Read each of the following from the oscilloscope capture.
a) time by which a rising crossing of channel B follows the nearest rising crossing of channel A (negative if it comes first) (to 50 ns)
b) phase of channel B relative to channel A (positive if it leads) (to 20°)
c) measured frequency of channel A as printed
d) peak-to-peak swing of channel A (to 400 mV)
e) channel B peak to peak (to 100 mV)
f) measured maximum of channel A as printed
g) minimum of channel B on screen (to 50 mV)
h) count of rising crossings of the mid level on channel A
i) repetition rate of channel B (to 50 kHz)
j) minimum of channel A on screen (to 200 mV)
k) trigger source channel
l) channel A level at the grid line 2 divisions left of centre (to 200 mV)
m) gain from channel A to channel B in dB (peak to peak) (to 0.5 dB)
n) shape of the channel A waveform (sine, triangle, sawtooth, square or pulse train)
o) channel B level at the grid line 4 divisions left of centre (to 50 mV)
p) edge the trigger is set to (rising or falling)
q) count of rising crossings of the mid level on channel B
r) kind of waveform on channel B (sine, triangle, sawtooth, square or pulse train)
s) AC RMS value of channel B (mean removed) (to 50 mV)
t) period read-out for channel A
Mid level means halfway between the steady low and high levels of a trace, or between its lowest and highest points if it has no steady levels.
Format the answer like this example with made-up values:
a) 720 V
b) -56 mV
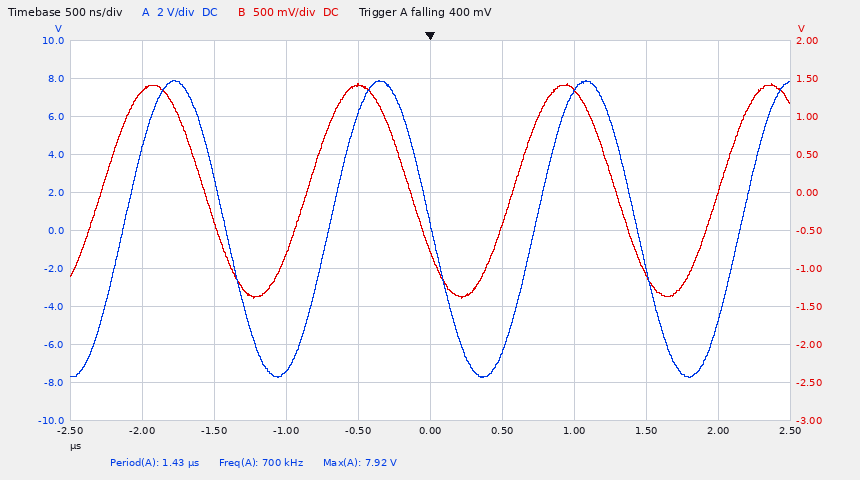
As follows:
a) -150 ns
b) +40°
c) 700 kHz
d) 15.6 V
e) 2.80 V
f) 7.92 V
g) -1.40 V
h) 4
i) 700 kHz
j) -7.8 V
k) channel A
l) -7.4 V
m) -15.0 dB
n) sine
o) 1.35 V
p) falling
q) 4
r) sine
s) 1.00 V
t) 1.43 µs
